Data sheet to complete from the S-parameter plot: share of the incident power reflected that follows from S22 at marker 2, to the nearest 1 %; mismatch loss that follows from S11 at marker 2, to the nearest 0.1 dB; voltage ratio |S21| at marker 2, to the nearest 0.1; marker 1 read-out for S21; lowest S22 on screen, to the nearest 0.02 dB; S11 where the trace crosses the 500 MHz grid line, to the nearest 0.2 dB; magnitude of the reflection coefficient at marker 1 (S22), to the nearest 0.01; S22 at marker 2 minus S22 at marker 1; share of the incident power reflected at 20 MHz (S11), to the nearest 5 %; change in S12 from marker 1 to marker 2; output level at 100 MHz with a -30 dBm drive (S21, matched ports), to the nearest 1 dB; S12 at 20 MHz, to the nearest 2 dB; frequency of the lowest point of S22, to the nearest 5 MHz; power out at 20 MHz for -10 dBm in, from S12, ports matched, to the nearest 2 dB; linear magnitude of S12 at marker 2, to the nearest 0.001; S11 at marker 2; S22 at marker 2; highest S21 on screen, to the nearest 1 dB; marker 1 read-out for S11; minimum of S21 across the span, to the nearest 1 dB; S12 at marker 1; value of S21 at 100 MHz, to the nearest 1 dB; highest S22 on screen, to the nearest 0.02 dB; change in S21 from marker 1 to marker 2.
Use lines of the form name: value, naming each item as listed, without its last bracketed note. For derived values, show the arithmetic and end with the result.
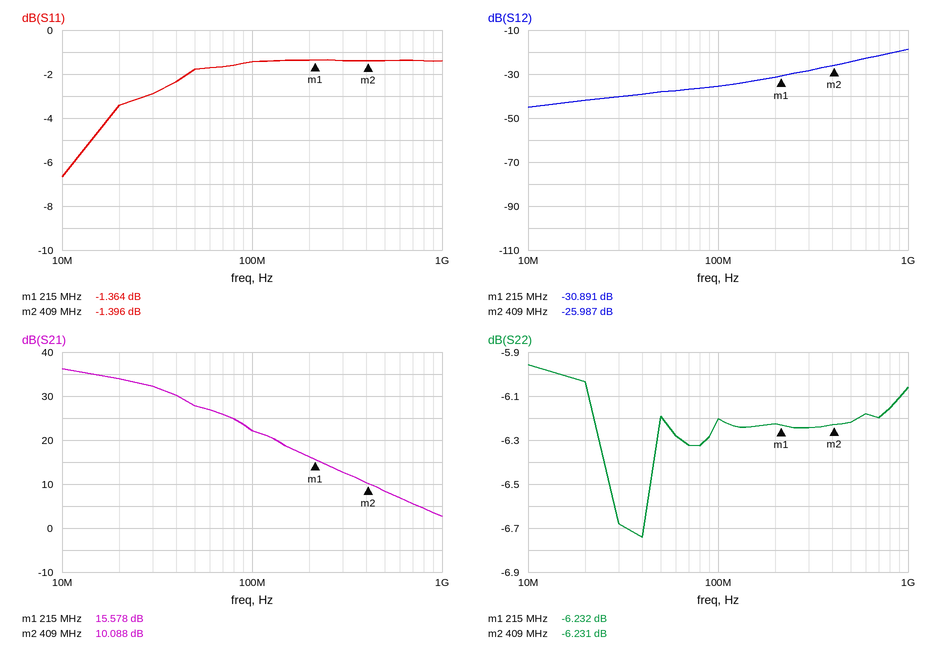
share of the incident power reflected that follows from S22 at marker 2, to the nearest 1 %: 10^(-6.231/10) ≈ 24 %
mismatch loss that follows from S11 at marker 2, to the nearest 0.1 dB: −10 log10(1 − 10^(-1.396/10)) ≈ 5.6 dB
voltage ratio |S21| at marker 2, to the nearest 0.1: 10^(10.088/20) ≈ 3.2
marker 1 read-out for S21: 15.578 dB
lowest S22 on screen, to the nearest 0.02 dB: -6.74 dB
S11 where the trace crosses the 500 MHz grid line, to the nearest 0.2 dB: -1.4 dB
magnitude of the reflection coefficient at marker 1 (S22), to the nearest 0.01: 10^(-6.232/20) ≈ 0.49
S22 at marker 2 minus S22 at marker 1: -6.231 − (-6.232) = 0.001 dB
share of the incident power reflected at 20 MHz (S11), to the nearest 5 %: 10^(-3.4/10) ≈ 45.7 %, so 45 % to the nearest 5 %
change in S12 from marker 1 to marker 2: -25.987 − (-30.891) = 4.904 dB
output level at 100 MHz with a -30 dBm drive (S21, matched ports), to the nearest 1 dB: -30 dBm + (22 dB) = -8 dBm
S12 at 20 MHz, to the nearest 2 dB: -42 dB
frequency of the lowest point of S22, to the nearest 5 MHz: 40 MHz
power out at 20 MHz for -10 dBm in, from S12, ports matched, to the nearest 2 dB: -10 dBm + (-42 dB) = -52 dBm
linear magnitude of S12 at marker 2, to the nearest 0.001: 10^(-25.987/20) ≈ 0.050
S11 at marker 2: -1.396 dB
S22 at marker 2: -6.231 dB
highest S21 on screen, to the nearest 1 dB: 36 dB
marker 1 read-out for S11: -1.364 dB
minimum of S21 across the span, to the nearest 1 dB: 3 dB
S12 at marker 1: -30.891 dB
value of S21 at 100 MHz, to the nearest 1 dB: 22 dB
highest S22 on screen, to the nearest 0.02 dB: -5.96 dB
change in S21 from marker 1 to marker 2: 10.088 − (15.578) = -5.490 dB
